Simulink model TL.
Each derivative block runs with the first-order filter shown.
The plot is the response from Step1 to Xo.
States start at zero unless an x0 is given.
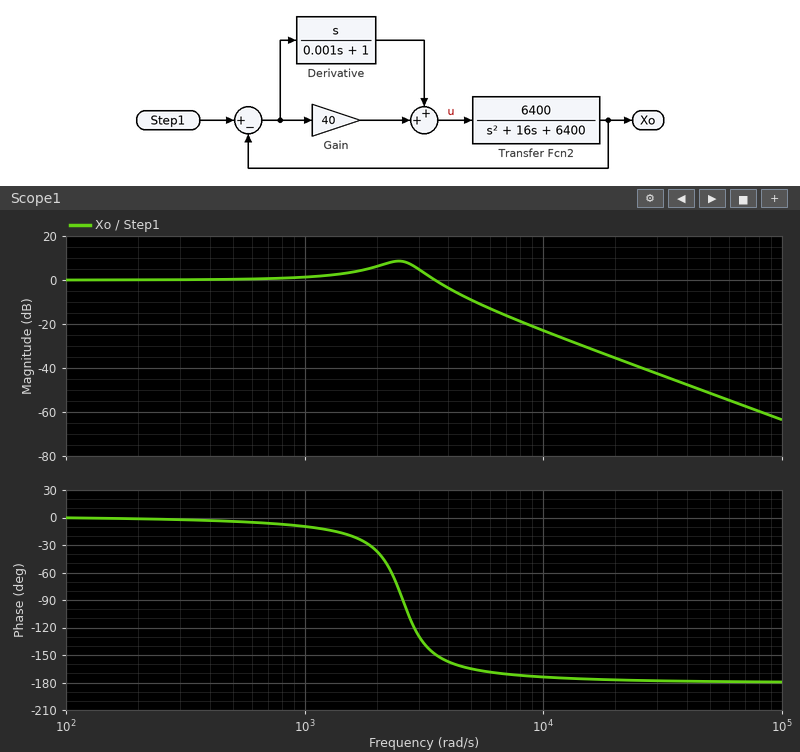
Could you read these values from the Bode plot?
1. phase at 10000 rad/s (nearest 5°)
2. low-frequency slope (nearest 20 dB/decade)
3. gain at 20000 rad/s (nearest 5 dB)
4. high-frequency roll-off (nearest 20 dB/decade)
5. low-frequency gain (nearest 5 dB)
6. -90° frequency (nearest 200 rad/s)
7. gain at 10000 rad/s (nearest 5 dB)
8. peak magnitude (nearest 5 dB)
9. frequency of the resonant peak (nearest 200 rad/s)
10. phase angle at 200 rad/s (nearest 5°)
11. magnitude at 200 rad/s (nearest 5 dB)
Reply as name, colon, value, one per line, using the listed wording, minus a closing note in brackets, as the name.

phase at 10000 rad/s: -175°
low-frequency slope: 0 dB/decade
gain at 20000 rad/s: -35 dB
high-frequency roll-off: -40 dB/decade
low-frequency gain: 0 dB
-90° frequency: 2600 rad/s
gain at 10000 rad/s: -25 dB
peak magnitude: 10 dB
frequency of the resonant peak: 2400 rad/s
phase angle at 200 rad/s: 0°
magnitude at 200 rad/s: 0 dB
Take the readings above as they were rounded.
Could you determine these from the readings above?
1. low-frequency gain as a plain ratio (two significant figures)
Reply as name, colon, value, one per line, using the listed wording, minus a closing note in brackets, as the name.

low-frequency gain as a plain ratio: 1.0
